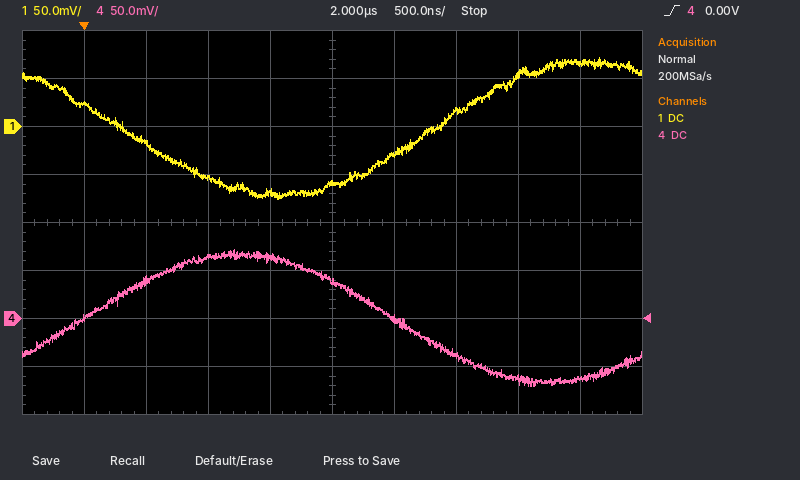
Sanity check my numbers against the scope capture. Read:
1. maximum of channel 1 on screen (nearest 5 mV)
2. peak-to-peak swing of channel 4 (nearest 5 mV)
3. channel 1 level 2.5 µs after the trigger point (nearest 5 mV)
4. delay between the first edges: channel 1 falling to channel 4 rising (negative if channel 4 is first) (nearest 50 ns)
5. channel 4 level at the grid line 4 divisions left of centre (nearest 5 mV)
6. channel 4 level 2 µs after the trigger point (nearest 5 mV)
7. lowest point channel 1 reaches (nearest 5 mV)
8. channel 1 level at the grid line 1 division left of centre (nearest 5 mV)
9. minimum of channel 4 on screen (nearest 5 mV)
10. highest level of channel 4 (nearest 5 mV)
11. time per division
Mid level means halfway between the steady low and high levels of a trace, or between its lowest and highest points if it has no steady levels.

70 mV
140 mV
-30 mV
-300 ns
0 mV
40 mV
-75 mV
-70 mV
-70 mV
70 mV
500 ns
